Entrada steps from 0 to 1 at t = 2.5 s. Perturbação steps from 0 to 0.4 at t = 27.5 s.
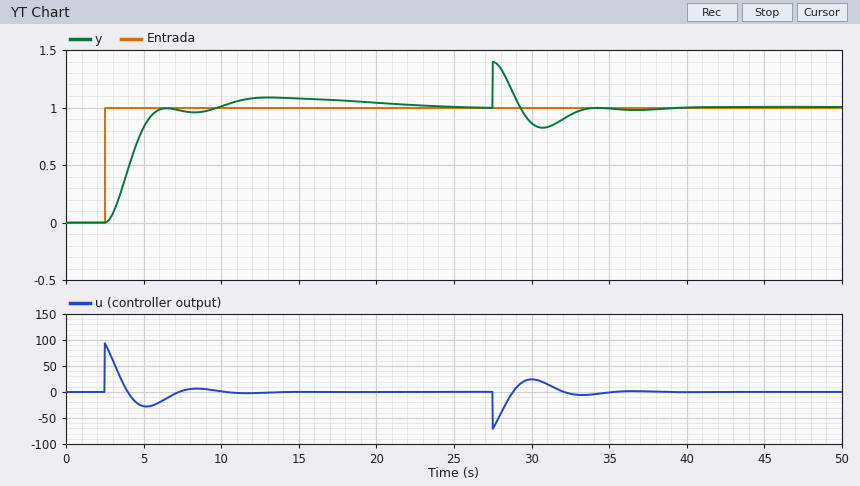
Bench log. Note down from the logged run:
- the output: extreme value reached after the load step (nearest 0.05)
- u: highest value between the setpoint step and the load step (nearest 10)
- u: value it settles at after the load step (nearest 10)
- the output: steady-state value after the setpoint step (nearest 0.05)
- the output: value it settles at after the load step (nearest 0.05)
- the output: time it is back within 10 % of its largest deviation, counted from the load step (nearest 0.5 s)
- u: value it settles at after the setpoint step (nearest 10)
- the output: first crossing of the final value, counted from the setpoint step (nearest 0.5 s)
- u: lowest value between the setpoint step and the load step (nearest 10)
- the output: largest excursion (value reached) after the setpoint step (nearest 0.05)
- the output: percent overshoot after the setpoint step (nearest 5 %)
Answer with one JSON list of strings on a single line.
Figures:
["1.40", "90", "0", "1.00", "1.00", "5.5 s", "0", "7.5 s", "-30", "1.10", "10 %"]
